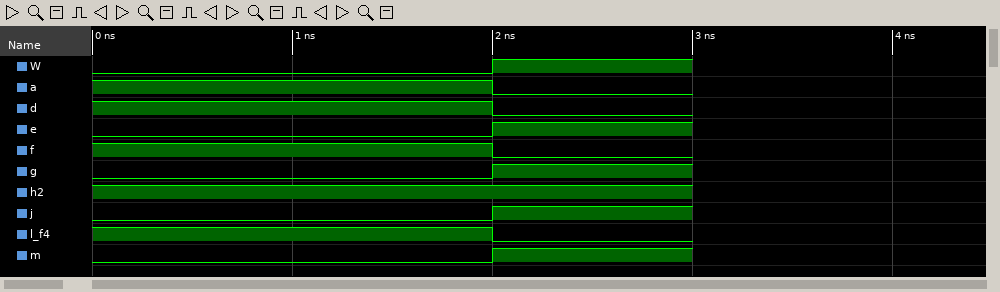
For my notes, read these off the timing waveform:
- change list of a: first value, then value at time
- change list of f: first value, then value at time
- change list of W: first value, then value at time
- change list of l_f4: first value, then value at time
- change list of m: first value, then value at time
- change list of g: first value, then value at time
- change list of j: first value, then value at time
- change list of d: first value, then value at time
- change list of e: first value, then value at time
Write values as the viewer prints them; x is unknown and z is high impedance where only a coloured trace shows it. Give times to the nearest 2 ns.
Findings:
1, 0 at 2 ns
1, 0 at 2 ns
0, 1 at 2 ns
1, 0 at 2 ns
0, 1 at 2 ns
0, 1 at 2 ns
0, 1 at 2 ns
1, 0 at 2 ns
0, 1 at 2 ns
